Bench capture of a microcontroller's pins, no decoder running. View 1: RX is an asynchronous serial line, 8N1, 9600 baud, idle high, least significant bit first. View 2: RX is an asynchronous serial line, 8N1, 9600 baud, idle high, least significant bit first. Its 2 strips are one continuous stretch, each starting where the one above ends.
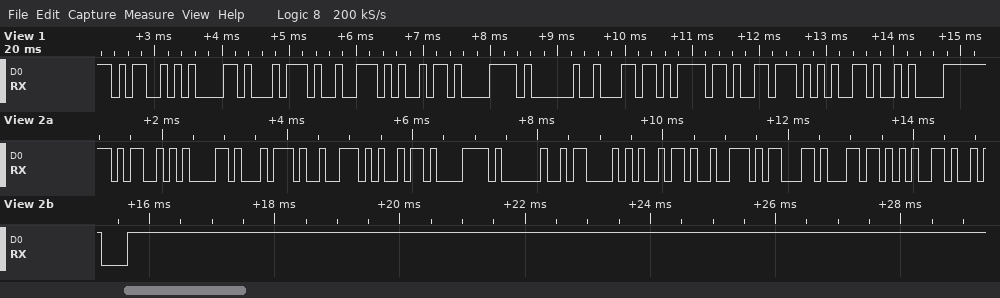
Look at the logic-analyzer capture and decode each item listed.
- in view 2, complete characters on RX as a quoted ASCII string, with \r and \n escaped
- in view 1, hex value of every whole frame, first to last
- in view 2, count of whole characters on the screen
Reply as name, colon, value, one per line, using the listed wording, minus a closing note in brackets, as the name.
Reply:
in view 2, complete characters on RX as a quoted ASCII string, with \r and \n escaped: "Matrix Circle\n"
in view 1, hex value of every whole frame, first to last: 4D 61 74 72 69 78 20 6C 6F 76 65 0A
in view 2, count of whole characters on the screen: 14
